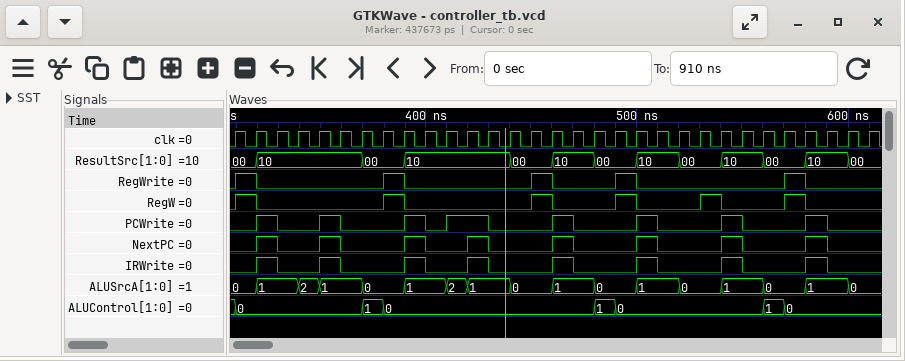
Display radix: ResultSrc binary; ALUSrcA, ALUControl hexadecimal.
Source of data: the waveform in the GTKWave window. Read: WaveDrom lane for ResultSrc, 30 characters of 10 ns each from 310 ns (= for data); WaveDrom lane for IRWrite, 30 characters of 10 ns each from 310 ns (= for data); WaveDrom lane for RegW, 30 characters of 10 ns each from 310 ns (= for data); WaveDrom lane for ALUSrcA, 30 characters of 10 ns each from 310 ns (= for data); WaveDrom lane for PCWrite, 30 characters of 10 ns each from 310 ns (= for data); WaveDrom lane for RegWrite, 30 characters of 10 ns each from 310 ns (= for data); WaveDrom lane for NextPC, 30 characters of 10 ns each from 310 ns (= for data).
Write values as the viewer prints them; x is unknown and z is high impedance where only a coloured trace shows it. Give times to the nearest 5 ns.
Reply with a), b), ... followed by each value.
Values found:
a) {name: 'ResultSrc', wave: '==....=.=....=.=.=.=.=.=.=.=.=', data: '00 10 00 10 00 10 00 10 00 10 00 10 00'}
b) {name: 'IRWrite', wave: '010.10..10.10..10..10..10..10.'}
c) {name: 'RegW', wave: '10.....10.....10..10..10..10..'}
d) {name: 'ALUSrcA', wave: '==.==.=.=.==.=.=.=.=.=.=.=.=.=', data: '0 1 2 1 0 1 2 1 0 1 0 1 0 1 0 1 0'}
e) {name: 'PCWrite', wave: '010.10..101.0..10..10..10..10.'}
f) {name: 'RegWrite', wave: '10.....10.....10..10......10..'}
g) {name: 'NextPC', wave: '010.10..10.10..10..10..10..10.'}
